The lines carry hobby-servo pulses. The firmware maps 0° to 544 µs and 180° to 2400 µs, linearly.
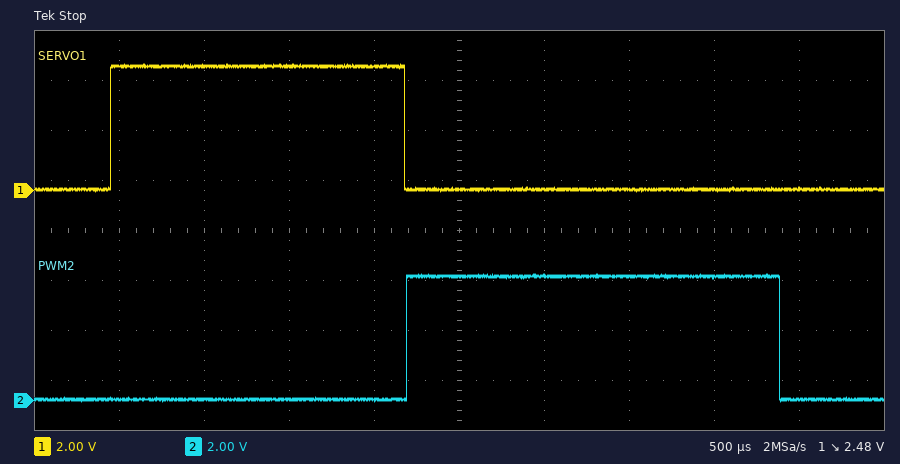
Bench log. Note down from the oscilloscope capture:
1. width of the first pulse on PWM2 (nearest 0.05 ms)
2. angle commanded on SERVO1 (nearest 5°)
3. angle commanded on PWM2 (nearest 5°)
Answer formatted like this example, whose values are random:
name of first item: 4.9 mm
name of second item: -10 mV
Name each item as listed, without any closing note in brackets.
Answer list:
width of the first pulse on PWM2: 2.20 ms
angle commanded on SERVO1: 115°
angle commanded on PWM2: 160°
